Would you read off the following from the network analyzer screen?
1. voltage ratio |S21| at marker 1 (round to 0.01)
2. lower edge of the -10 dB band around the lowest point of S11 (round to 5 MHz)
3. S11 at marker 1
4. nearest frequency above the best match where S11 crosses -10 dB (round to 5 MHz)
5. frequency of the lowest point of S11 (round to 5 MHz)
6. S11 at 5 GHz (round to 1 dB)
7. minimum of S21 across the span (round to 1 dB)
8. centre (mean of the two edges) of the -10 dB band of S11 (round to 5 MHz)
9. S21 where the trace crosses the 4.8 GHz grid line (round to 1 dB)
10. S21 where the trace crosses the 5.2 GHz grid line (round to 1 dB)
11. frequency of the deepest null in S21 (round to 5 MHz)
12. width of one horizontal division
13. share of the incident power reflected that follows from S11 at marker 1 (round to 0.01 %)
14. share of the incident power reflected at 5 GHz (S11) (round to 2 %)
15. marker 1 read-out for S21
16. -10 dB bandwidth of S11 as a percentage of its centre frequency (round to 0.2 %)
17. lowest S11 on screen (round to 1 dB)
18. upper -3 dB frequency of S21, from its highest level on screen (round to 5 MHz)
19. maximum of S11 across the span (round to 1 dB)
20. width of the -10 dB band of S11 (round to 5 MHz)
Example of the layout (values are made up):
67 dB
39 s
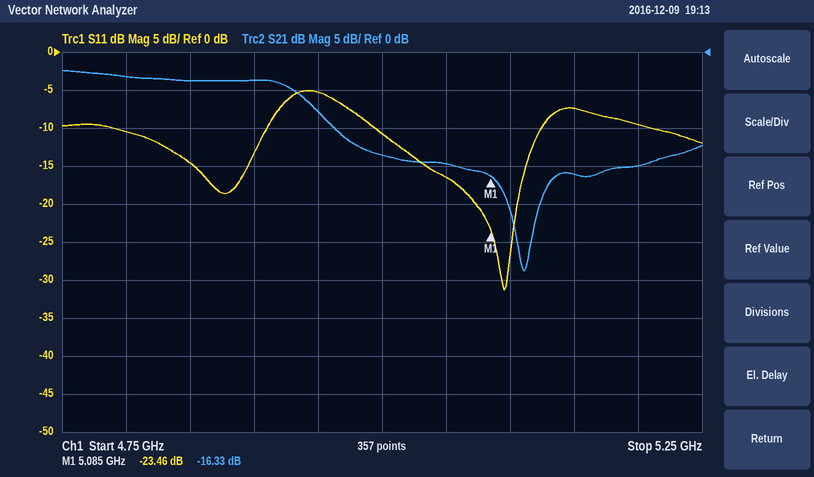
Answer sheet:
0.15
4.995 GHz
-23.46 dB
5.125 GHz
5.095 GHz
-11 dB
-29 dB
5.060 GHz
-3 dB
-15 dB
5.110 GHz
50 MHz
0.45 %
8 %
-16.33 dB
2.6 %
-31 dB
4.935 GHz
-5 dB
130 MHz
